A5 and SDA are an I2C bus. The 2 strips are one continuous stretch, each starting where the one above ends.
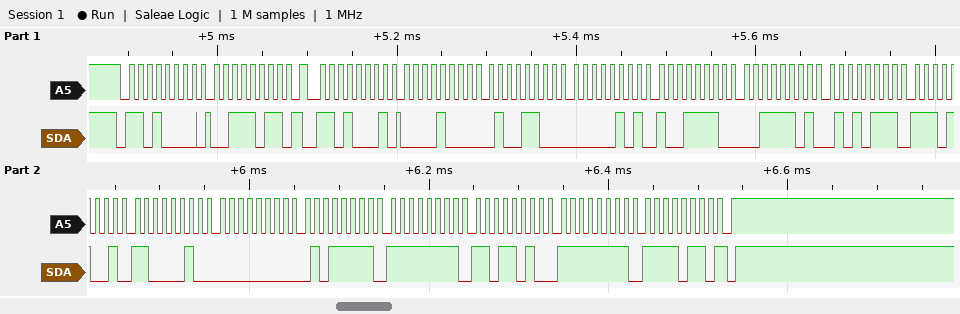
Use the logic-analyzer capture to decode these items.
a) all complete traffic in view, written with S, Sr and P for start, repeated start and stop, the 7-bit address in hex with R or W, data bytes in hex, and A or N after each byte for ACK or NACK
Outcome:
S 68W A 3B A Sr 68R A 08 A 4C A 05 A 9E A 3D A 57 A E9 A C2 A 00 A 5F A FF A DA A FF A F6 N P
